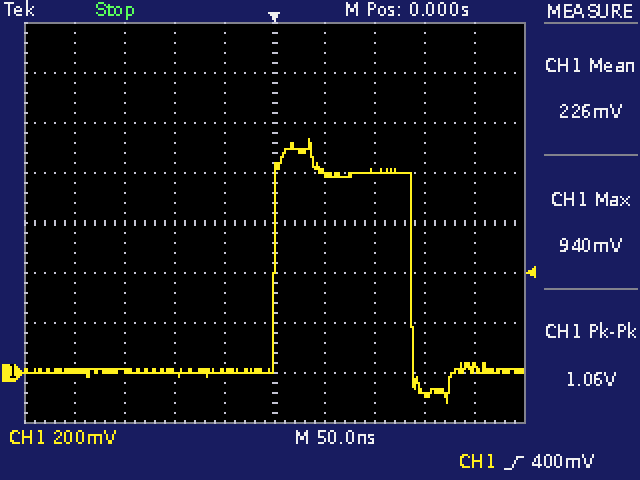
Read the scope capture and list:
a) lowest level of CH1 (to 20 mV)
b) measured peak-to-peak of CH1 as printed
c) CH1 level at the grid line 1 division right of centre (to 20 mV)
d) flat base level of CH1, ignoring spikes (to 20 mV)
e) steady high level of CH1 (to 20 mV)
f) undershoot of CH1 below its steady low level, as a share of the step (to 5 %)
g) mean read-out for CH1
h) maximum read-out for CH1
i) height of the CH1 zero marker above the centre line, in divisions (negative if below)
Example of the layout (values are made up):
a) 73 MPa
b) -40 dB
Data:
a) -120 mV
b) 1.06 V
c) 800 mV
d) 0 mV
e) 800 mV
f) 15 %
g) 226 mV
h) 940 mV
i) -3.0 div
